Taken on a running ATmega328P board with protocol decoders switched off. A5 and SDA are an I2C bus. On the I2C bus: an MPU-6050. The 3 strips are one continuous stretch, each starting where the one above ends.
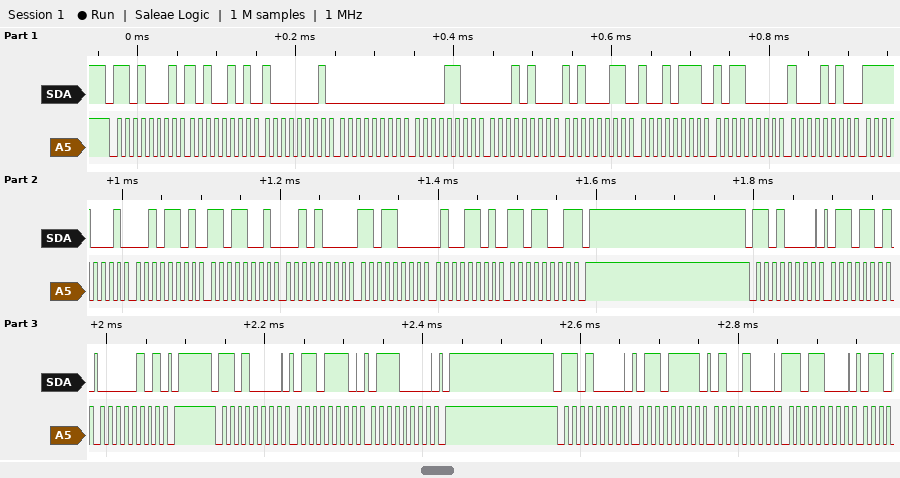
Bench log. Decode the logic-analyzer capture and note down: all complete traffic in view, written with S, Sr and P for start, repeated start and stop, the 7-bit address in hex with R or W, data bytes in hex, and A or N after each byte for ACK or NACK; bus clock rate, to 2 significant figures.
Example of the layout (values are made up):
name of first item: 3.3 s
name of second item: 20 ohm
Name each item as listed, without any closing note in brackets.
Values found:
all complete traffic in view, written with S, Sr and P for start, repeated start and stop, the 7-bit address in hex with R or W, data bytes in hex, and A or N after each byte for ACK or NACK: S 68R A A5 A 81 A 00 A 0C A 14 A A3 A 97 A B0 A 8A A F1 A 2D A D9 A 28 A D8 A 4D A D9 N P S 68W A 6D A 05 A P S 68W A 6E A 70 A P S 68W A 6F A 48 A D8 A
bus clock rate, to 2 significant figures: 100 kHz
